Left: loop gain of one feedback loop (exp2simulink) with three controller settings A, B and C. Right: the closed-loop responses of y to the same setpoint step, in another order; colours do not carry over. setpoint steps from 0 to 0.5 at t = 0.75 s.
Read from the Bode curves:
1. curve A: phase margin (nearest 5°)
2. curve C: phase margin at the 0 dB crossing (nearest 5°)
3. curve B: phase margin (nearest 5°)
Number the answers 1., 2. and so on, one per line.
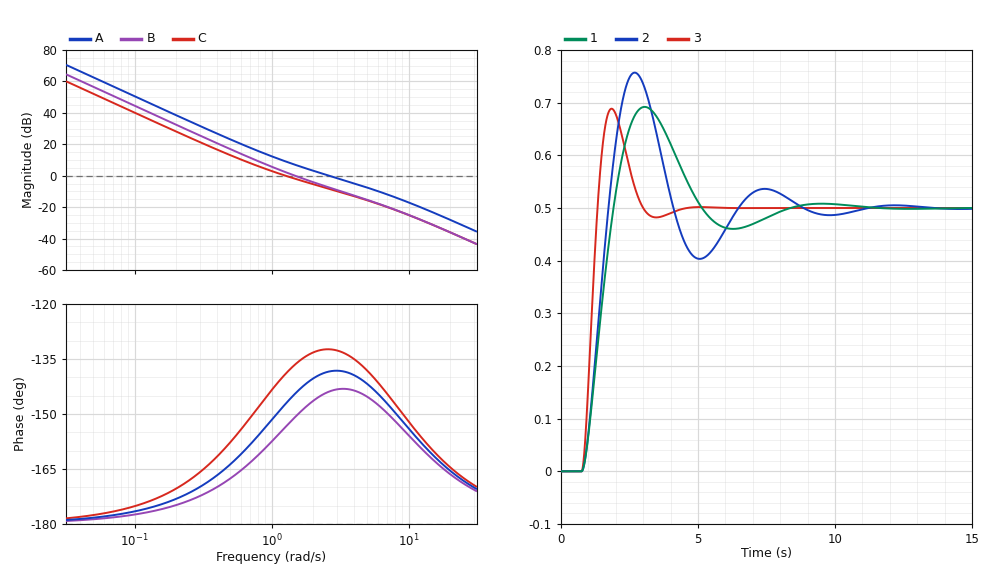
1. 40°
2. 40°
3. 30°
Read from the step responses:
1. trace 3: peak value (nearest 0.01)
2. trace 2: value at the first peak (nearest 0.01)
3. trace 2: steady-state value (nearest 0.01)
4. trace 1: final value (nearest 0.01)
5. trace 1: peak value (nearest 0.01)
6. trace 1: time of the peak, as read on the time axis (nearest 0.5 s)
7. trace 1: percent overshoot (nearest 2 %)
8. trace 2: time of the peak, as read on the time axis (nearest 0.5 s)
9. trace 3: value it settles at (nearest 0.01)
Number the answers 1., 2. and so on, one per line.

1. 0.69
2. 0.76
3. 0.50
4. 0.50
5. 0.69
6. 3.0 s
7. 38 %
8. 2.5 s
9. 0.50
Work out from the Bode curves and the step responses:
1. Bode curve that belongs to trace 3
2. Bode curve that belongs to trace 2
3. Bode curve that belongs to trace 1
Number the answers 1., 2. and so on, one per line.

1. A
2. B
3. C
